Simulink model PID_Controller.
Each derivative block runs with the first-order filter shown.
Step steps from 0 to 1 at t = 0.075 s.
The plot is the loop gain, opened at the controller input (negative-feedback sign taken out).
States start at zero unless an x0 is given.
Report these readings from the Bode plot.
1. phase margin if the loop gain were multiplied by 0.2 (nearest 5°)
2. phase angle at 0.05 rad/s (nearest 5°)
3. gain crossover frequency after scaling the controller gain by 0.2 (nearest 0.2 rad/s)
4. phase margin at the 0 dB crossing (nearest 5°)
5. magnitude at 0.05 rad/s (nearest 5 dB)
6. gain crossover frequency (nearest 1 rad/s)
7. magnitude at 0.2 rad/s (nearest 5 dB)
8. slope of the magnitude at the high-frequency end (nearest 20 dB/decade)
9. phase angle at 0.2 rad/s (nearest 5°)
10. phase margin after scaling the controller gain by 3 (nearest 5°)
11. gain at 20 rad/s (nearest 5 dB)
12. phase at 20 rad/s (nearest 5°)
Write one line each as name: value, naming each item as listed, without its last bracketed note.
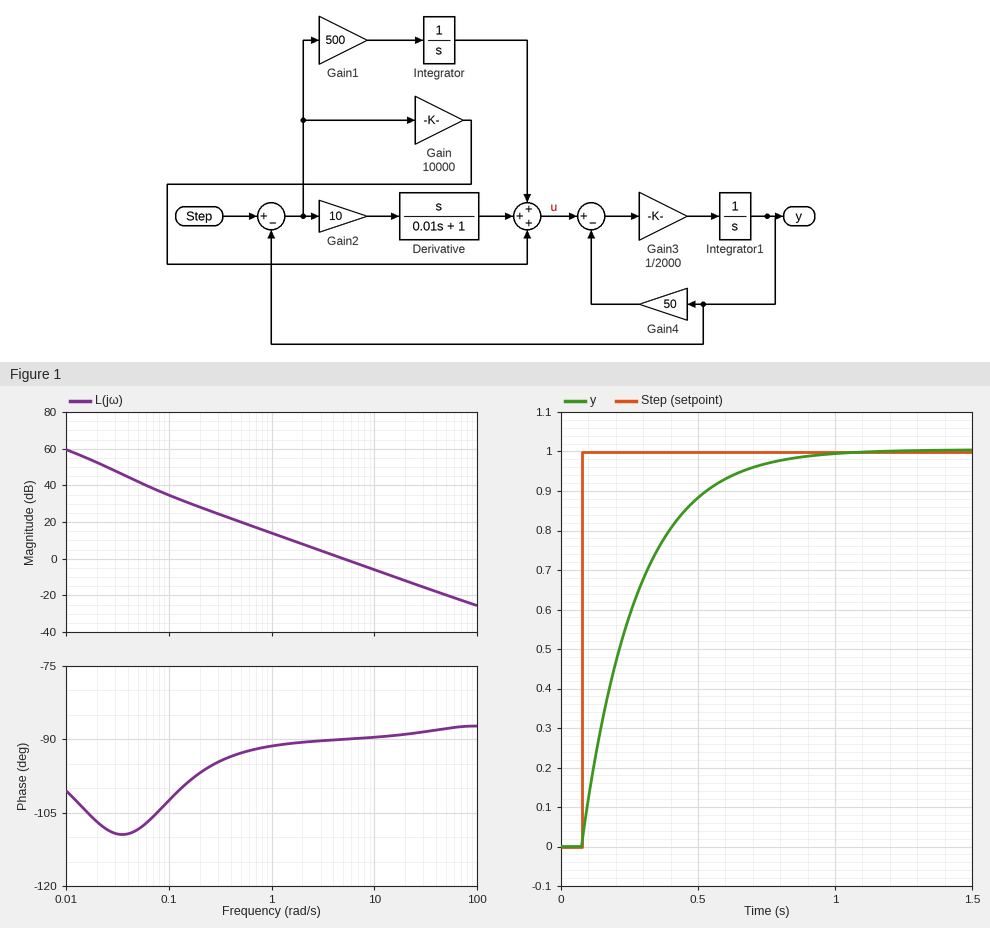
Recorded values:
phase margin if the loop gain were multiplied by 0.2: 90°
phase angle at 0.05 rad/s: -110°
gain crossover frequency after scaling the controller gain by 0.2: 1.0 rad/s
phase margin at the 0 dB crossing: 90°
magnitude at 0.05 rad/s: 40 dB
gain crossover frequency: 5 rad/s
magnitude at 0.2 rad/s: 30 dB
slope of the magnitude at the high-frequency end: -20 dB/decade
phase angle at 0.2 rad/s: -95°
phase margin after scaling the controller gain by 3: 90°
gain at 20 rad/s: -10 dB
phase at 20 rad/s: -90°
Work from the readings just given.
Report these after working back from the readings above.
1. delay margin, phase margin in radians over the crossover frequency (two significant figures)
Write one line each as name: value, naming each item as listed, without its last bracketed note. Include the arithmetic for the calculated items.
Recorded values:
delay margin, phase margin in radians over the crossover frequency: 90 × π / 180 / 5 = 0.31 s
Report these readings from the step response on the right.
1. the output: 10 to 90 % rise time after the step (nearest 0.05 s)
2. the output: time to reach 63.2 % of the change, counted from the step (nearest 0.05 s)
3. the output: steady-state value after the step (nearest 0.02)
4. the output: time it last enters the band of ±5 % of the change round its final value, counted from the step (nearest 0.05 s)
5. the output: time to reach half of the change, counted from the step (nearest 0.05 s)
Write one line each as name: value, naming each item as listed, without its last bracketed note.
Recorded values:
the output: 10 to 90 % rise time after the step: 0.45 s
the output: time to reach 63.2 % of the change, counted from the step: 0.20 s
the output: steady-state value after the step: 1.00
the output: time it last enters the band of ±5 % of the change round its final value, counted from the step: 0.60 s
the output: time to reach half of the change, counted from the step: 0.15 s
